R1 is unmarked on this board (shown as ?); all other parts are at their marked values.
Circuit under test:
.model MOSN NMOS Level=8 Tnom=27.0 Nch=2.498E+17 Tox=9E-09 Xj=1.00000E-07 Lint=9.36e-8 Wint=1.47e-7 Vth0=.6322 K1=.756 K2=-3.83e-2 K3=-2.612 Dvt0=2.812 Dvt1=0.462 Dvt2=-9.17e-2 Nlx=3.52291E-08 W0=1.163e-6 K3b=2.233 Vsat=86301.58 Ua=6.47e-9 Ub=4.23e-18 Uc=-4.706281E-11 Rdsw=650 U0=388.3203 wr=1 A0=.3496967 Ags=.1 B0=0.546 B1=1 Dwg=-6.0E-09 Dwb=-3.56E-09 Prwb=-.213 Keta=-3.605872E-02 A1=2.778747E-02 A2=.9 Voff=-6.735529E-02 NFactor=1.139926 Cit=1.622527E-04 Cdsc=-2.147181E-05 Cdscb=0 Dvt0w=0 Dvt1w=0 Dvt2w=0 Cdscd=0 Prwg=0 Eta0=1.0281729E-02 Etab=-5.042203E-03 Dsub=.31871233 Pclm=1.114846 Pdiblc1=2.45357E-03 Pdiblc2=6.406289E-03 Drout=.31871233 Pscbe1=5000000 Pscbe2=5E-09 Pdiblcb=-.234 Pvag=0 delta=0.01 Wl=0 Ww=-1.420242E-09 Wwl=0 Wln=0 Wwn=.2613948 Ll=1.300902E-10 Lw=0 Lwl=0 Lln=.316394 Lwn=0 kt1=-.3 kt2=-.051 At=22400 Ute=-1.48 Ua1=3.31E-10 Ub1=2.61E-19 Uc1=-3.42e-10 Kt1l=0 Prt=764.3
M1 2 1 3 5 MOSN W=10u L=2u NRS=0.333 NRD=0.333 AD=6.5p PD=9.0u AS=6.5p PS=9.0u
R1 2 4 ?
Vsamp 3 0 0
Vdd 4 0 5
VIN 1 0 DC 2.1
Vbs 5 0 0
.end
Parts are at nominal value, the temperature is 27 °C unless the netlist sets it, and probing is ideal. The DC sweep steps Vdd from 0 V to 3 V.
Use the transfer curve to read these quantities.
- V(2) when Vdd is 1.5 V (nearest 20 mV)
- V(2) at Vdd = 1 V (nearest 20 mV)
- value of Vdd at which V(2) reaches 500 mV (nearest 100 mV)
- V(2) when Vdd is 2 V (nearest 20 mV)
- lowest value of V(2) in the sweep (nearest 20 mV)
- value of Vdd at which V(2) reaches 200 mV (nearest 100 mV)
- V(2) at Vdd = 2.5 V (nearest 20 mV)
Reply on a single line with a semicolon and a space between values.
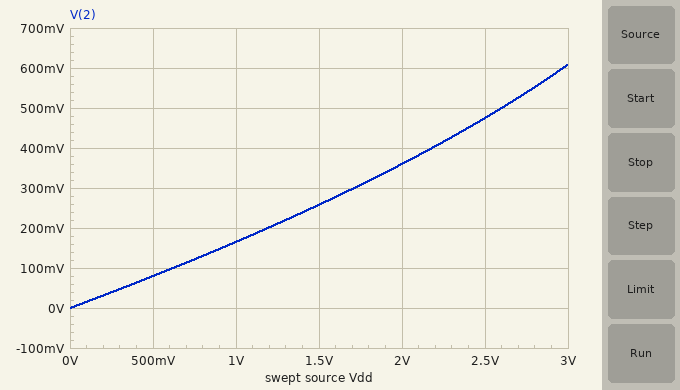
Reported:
260 mV; 160 mV; 2.6 V; 360 mV; 0 V; 1.2 V; 480 mV
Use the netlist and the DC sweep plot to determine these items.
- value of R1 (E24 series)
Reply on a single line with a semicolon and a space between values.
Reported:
16 kΩ
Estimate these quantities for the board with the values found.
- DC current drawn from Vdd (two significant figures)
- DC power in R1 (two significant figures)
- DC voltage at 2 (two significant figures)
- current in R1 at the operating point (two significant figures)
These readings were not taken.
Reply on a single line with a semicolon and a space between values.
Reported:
190 µA; 600 µW; 1.9 V; 190 µA
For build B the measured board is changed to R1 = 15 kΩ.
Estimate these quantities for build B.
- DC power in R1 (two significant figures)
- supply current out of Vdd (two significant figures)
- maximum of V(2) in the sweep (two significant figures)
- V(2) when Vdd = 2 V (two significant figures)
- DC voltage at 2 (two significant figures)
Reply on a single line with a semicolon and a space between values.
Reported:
570 µW; 190 µA; 660 mV; 380 mV; 2.1 V
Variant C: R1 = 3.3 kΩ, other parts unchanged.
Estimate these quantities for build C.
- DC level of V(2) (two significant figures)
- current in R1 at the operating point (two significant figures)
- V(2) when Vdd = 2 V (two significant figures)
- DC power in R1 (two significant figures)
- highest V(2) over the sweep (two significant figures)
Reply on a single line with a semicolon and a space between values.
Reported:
4.3 V; 200 µA; 1.4 V; 130 µW; 2.4 V
